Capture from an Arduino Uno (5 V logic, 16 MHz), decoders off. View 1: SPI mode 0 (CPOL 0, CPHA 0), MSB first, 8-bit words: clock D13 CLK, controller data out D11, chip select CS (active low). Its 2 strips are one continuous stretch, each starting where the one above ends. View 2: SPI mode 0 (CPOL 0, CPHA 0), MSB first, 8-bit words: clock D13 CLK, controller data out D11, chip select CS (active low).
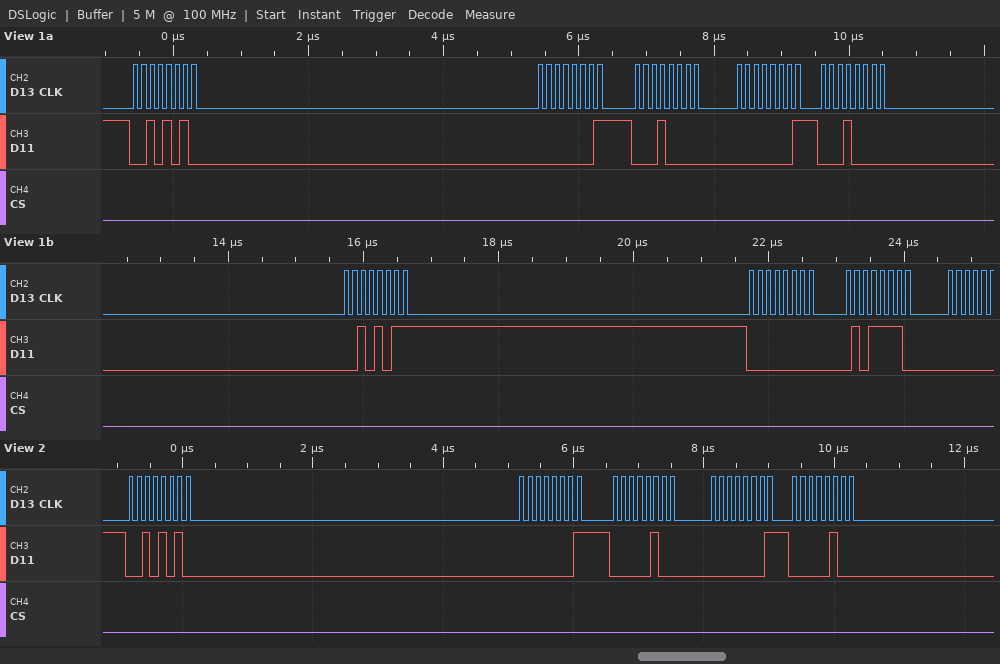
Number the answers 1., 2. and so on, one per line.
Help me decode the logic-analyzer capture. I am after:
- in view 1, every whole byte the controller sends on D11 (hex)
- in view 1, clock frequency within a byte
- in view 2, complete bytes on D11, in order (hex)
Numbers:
1. 0x2A 0x01 0x10 0x01 0x10 0x2B 0x00 0x5E
2. 8 MHz
3. 2A 01 04 01 04
